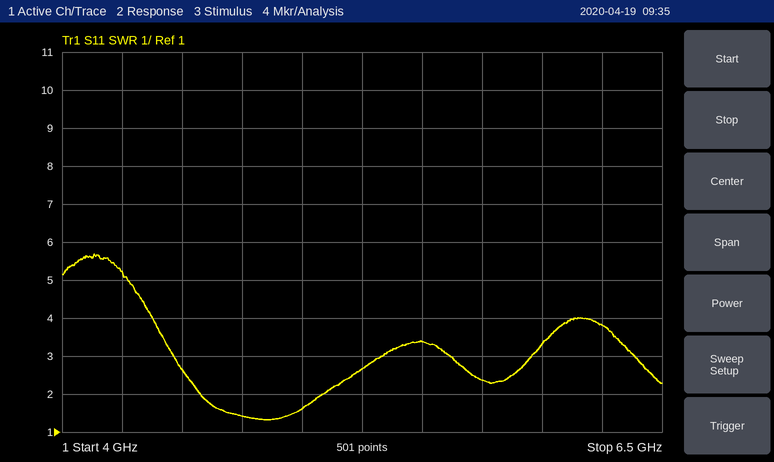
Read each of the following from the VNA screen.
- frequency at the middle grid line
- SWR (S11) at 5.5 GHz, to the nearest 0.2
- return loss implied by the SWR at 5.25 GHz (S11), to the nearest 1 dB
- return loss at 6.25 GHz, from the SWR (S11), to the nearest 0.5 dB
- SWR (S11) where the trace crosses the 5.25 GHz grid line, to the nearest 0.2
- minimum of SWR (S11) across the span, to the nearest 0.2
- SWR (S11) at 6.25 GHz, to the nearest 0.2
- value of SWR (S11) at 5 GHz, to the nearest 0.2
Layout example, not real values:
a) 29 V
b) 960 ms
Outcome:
a) 5.25 GHz
b) 3.4
c) 7 dB
d) 4.5 dB
e) 2.6
f) 1.4
g) 3.8
h) 1.6
